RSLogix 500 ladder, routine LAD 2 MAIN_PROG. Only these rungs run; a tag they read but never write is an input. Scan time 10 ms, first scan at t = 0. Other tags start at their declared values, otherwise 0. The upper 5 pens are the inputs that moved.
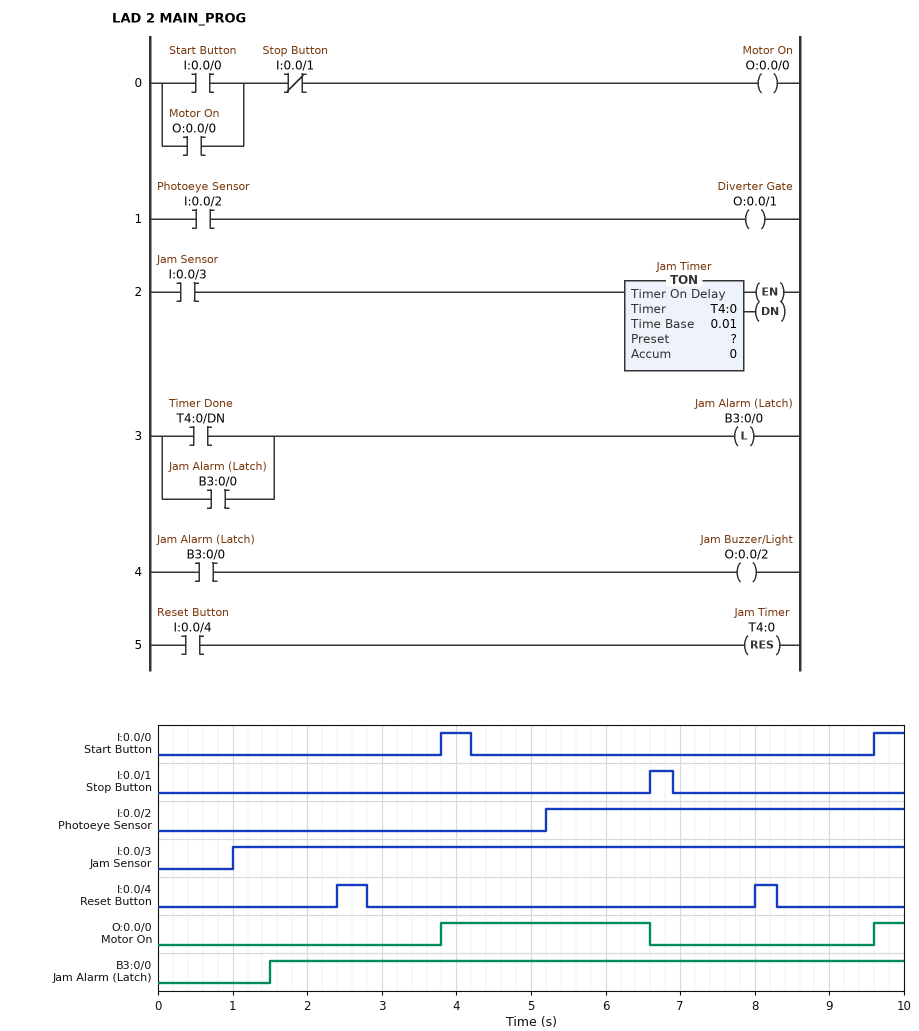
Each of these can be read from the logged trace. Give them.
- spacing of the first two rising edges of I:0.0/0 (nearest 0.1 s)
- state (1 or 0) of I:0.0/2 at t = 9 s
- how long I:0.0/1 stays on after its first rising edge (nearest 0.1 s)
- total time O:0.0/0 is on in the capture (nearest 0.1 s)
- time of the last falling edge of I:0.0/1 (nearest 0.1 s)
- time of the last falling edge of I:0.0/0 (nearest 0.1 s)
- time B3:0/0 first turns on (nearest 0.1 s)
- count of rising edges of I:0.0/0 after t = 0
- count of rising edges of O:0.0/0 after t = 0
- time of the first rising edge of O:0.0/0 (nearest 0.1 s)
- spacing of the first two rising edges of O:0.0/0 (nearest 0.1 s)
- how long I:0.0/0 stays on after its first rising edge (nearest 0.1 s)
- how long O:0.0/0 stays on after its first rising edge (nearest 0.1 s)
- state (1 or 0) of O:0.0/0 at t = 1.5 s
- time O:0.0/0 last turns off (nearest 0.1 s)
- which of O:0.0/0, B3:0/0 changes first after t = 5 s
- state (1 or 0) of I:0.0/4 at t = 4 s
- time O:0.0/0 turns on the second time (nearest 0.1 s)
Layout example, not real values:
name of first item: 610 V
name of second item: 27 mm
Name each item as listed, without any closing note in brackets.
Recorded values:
spacing of the first two rising edges of I:0.0/0: 5.8 s
state (1 or 0) of I:0.0/2 at t = 9 s: 1
how long I:0.0/1 stays on after its first rising edge: 0.3 s
total time O:0.0/0 is on in the capture: 3.2 s
time of the last falling edge of I:0.0/1: 6.9 s
time of the last falling edge of I:0.0/0: 4.2 s
time B3:0/0 first turns on: 1.5 s
count of rising edges of I:0.0/0 after t = 0: 2
count of rising edges of O:0.0/0 after t = 0: 2
time of the first rising edge of O:0.0/0: 3.8 s
spacing of the first two rising edges of O:0.0/0: 5.8 s
how long I:0.0/0 stays on after its first rising edge: 0.4 s
how long O:0.0/0 stays on after its first rising edge: 2.8 s
state (1 or 0) of O:0.0/0 at t = 1.5 s: 0
time O:0.0/0 last turns off: 6.6 s
which of O:0.0/0, B3:0/0 changes first after t = 5 s: O:0.0/0
state (1 or 0) of I:0.0/4 at t = 4 s: 0
time O:0.0/0 turns on the second time: 9.6 s
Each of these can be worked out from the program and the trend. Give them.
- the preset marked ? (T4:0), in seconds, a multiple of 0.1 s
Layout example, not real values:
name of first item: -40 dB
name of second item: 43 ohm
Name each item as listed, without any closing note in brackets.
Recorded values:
the preset marked ? (T4:0), in seconds, a multiple of 0.1 s: 0.5 s
